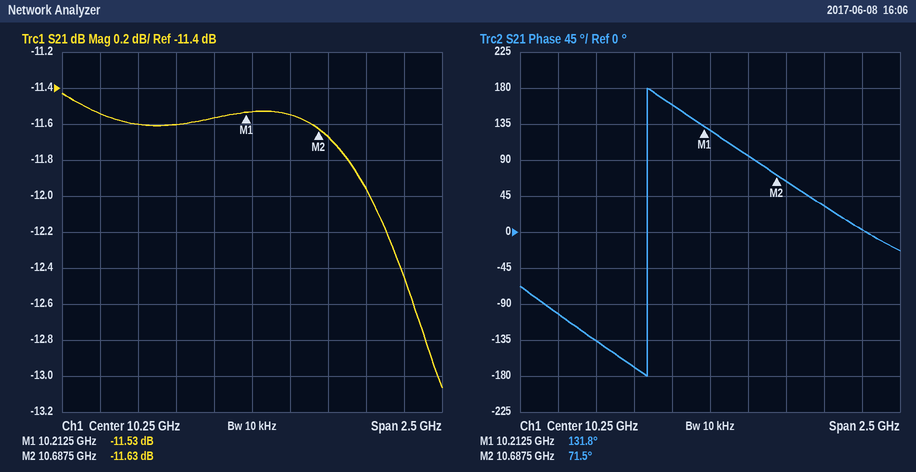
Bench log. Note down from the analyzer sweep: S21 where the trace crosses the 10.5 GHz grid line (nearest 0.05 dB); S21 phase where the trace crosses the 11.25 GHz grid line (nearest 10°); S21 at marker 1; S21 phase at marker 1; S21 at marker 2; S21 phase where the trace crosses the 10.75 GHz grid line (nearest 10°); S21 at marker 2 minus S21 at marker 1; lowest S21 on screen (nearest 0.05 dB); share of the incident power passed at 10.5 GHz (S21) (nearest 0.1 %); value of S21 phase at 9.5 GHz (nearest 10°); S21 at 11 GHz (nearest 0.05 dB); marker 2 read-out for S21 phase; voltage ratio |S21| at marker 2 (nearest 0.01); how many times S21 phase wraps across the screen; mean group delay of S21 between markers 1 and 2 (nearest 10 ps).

-11.55 dB
0°
-11.53 dB
131.8°
-11.63 dB
60°
-0.10 dB
-13.05 dB
7.0 %
-140°
-11.95 dB
71.5°
0.26
1
350 ps
